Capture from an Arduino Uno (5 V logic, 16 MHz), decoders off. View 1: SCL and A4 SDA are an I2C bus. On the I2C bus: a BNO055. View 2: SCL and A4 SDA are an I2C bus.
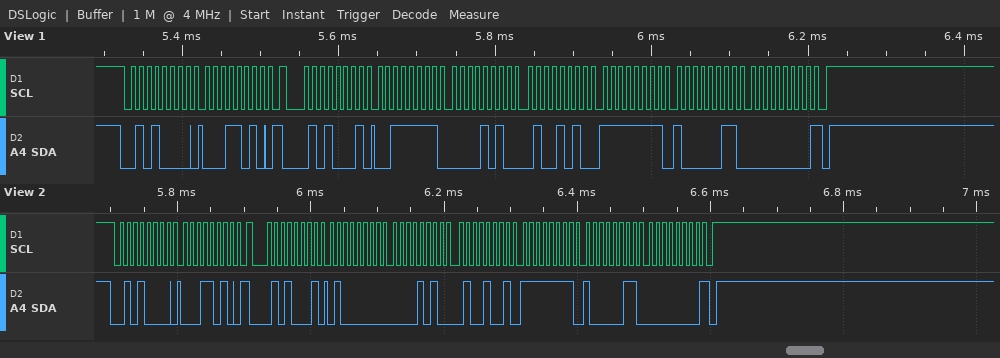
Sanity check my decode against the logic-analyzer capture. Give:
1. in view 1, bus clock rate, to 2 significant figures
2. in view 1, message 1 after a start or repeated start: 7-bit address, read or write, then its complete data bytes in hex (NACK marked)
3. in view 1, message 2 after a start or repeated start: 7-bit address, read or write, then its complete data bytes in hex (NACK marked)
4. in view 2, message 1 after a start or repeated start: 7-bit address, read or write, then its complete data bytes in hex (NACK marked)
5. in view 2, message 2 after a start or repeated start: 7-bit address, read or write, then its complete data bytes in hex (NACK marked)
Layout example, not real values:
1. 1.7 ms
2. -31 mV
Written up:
1. 100 kHz
2. 0x28 write: 1A
3. 0x28 read: 3F 0A 4A FF 83 00 NACK
4. 0x28 write: 1A
5. 0x28 read: 40 0A 49 FF 83 00 NACK
